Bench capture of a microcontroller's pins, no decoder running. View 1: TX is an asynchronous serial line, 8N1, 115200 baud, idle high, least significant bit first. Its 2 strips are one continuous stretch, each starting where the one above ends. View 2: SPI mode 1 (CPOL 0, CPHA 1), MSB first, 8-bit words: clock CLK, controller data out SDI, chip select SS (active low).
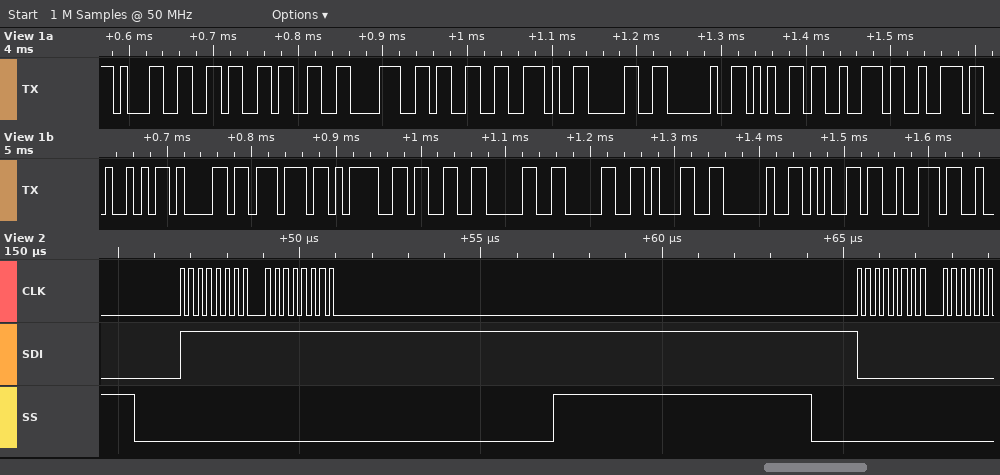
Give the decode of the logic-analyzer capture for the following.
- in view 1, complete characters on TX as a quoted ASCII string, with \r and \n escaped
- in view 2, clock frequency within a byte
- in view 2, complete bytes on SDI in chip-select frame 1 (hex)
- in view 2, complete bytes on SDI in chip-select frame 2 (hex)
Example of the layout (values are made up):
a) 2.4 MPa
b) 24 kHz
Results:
a) "16383.0 errRaw=3001 er"
b) 4 MHz
c) FF FF
d) 00
